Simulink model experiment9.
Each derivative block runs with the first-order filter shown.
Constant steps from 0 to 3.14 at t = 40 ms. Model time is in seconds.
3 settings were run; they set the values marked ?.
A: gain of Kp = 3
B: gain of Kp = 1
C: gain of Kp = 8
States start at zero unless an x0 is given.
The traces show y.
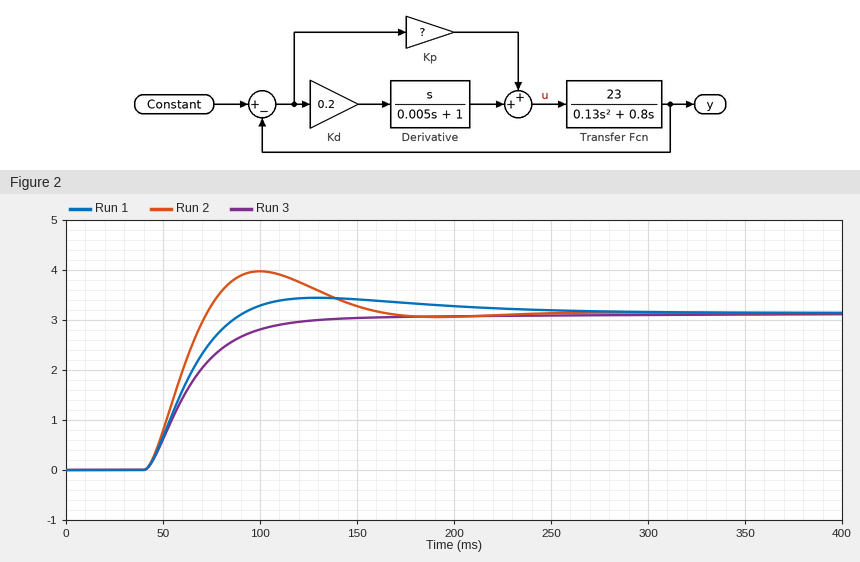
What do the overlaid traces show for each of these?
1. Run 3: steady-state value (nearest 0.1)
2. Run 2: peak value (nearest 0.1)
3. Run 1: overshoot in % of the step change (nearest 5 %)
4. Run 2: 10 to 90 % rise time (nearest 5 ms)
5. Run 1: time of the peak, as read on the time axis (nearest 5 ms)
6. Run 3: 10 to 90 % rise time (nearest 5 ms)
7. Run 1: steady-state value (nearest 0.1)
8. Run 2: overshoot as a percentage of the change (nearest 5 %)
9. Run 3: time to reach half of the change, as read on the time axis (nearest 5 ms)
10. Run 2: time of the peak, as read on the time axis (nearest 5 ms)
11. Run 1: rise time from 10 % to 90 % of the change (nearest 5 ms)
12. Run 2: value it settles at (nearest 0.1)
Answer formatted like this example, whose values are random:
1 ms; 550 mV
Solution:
3.1; 4.0; 10 %; 25 ms; 130 ms; 55 ms; 3.1; 25 %; 60 ms; 100 ms; 35 ms; 3.1
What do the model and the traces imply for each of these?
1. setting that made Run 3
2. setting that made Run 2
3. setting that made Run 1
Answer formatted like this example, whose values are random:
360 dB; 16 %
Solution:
B; C; A
